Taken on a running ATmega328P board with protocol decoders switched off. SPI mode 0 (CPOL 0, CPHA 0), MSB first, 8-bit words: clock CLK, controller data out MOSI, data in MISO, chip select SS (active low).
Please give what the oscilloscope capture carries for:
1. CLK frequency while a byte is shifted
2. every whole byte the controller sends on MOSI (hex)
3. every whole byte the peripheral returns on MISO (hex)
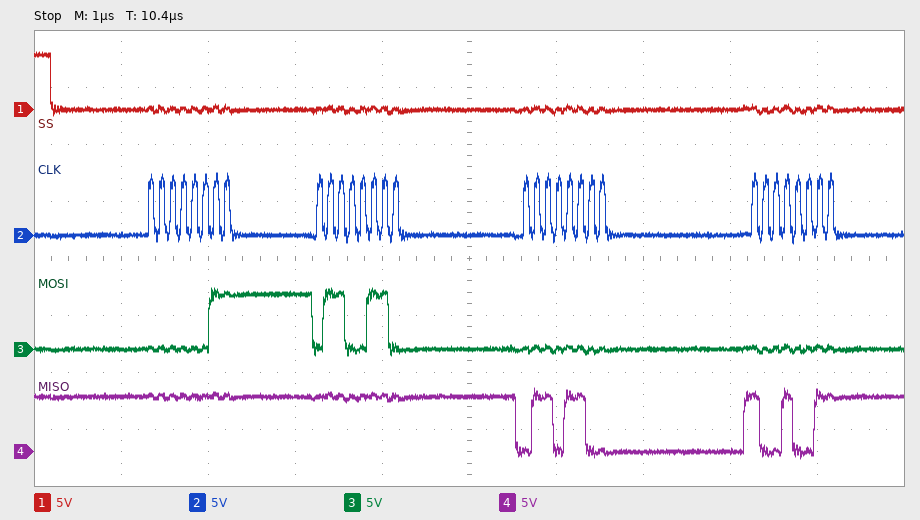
8 MHz
0x03 0x66 0x00 0x00
0xFF 0xFF 0x6C 0x93
